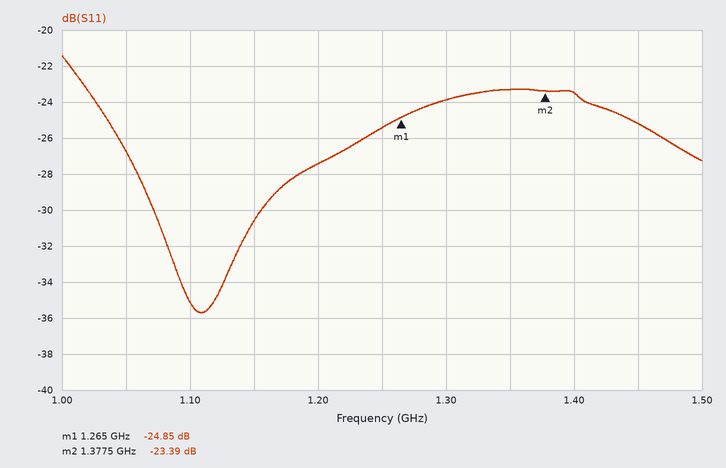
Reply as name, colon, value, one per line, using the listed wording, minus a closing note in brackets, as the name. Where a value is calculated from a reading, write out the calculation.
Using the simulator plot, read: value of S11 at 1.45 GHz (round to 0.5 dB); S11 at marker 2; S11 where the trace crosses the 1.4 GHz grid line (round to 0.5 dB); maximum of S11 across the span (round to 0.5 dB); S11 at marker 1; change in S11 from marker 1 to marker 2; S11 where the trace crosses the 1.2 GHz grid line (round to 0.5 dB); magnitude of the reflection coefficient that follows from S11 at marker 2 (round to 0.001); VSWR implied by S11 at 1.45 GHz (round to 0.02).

value of S11 at 1.45 GHz: -25.0 dB
S11 at marker 2: -23.39 dB
S11 where the trace crosses the 1.4 GHz grid line: -23.5 dB
maximum of S11 across the span: -21.5 dB
S11 at marker 1: -24.85 dB
change in S11 from marker 1 to marker 2: -23.39 − (-24.85) = 1.46 dB
S11 where the trace crosses the 1.2 GHz grid line: -27.5 dB
magnitude of the reflection coefficient that follows from S11 at marker 2: 10^(-23.39/20) ≈ 0.068
VSWR implied by S11 at 1.45 GHz: |Γ| = 10^(-25/20) = 0.0562; VSWR = (1 + 0.0562)/(1 − 0.0562) ≈ 1.12
